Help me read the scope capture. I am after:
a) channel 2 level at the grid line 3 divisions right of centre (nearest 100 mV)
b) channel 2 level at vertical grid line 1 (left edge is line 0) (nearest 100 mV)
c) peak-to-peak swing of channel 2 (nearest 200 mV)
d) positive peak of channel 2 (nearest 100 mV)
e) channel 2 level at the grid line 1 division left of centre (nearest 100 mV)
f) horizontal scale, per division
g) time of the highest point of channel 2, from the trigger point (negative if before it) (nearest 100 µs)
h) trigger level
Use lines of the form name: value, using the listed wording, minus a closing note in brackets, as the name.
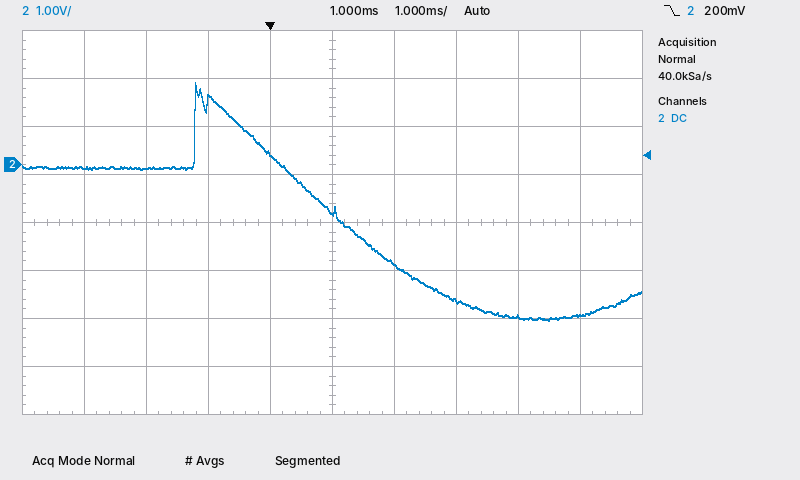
channel 2 level at the grid line 3 divisions right of centre: -3.2 V
channel 2 level at vertical grid line 1 (left edge is line 0): -100 mV
peak-to-peak swing of channel 2: 5.0 V
positive peak of channel 2: 1.7 V
channel 2 level at the grid line 1 division left of centre: 200 mV
horizontal scale, per division: 1 ms
time of the highest point of channel 2, from the trigger point (negative if before it): -1.2 ms
trigger level: 200 mV
